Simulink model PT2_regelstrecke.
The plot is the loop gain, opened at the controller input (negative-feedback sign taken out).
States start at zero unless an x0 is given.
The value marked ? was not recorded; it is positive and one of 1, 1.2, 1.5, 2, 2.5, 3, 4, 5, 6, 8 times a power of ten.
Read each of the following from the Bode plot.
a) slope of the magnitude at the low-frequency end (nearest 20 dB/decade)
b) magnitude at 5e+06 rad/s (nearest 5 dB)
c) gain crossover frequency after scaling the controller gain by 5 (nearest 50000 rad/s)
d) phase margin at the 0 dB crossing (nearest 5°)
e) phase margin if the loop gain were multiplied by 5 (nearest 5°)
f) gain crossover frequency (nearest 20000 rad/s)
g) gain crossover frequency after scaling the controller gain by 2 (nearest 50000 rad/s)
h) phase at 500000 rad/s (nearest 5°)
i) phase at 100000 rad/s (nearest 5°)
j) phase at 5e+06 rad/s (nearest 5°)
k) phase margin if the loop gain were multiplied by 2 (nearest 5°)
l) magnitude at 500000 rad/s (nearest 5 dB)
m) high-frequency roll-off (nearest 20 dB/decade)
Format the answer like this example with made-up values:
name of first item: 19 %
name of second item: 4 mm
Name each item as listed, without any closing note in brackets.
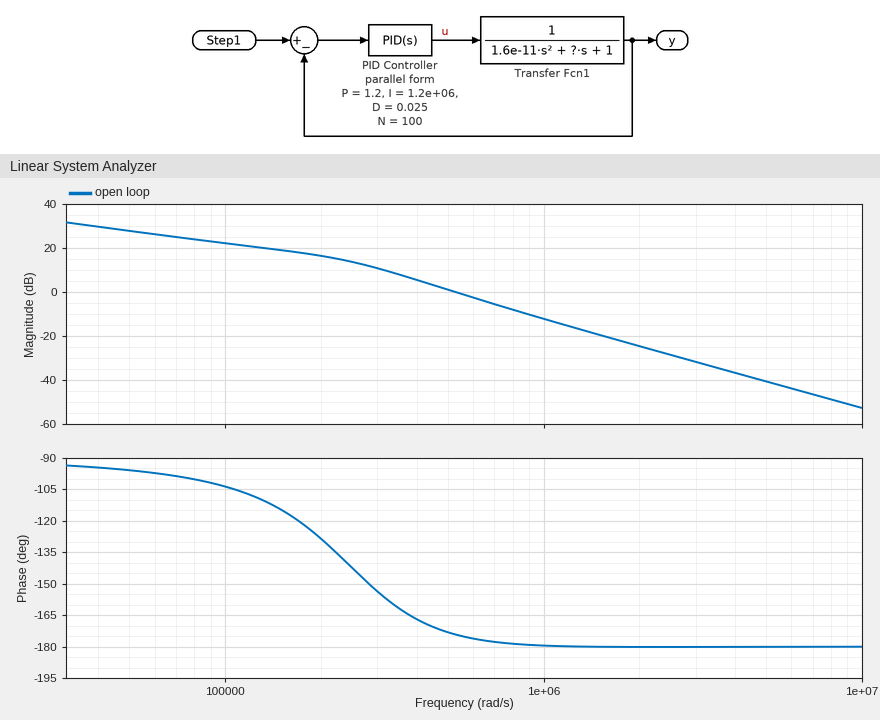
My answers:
slope of the magnitude at the low-frequency end: -20 dB/decade
magnitude at 5e+06 rad/s: -40 dB
gain crossover frequency after scaling the controller gain by 5: 1100000 rad/s
phase margin at the 0 dB crossing: 5°
phase margin if the loop gain were multiplied by 5: 0°
gain crossover frequency: 520000 rad/s
gain crossover frequency after scaling the controller gain by 2: 700000 rad/s
phase at 500000 rad/s: -175°
phase at 100000 rad/s: -105°
phase at 5e+06 rad/s: -180°
phase margin if the loop gain were multiplied by 2: 0°
magnitude at 500000 rad/s: 0 dB
high-frequency roll-off: -40 dB/decade
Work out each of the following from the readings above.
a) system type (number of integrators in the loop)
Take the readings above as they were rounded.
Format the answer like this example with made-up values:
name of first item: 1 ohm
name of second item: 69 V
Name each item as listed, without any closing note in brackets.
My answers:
system type: 1
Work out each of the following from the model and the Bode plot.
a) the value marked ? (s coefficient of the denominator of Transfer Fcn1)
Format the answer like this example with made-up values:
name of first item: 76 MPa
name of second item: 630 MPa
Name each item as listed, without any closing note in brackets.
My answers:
the value marked ?: 5e-06
